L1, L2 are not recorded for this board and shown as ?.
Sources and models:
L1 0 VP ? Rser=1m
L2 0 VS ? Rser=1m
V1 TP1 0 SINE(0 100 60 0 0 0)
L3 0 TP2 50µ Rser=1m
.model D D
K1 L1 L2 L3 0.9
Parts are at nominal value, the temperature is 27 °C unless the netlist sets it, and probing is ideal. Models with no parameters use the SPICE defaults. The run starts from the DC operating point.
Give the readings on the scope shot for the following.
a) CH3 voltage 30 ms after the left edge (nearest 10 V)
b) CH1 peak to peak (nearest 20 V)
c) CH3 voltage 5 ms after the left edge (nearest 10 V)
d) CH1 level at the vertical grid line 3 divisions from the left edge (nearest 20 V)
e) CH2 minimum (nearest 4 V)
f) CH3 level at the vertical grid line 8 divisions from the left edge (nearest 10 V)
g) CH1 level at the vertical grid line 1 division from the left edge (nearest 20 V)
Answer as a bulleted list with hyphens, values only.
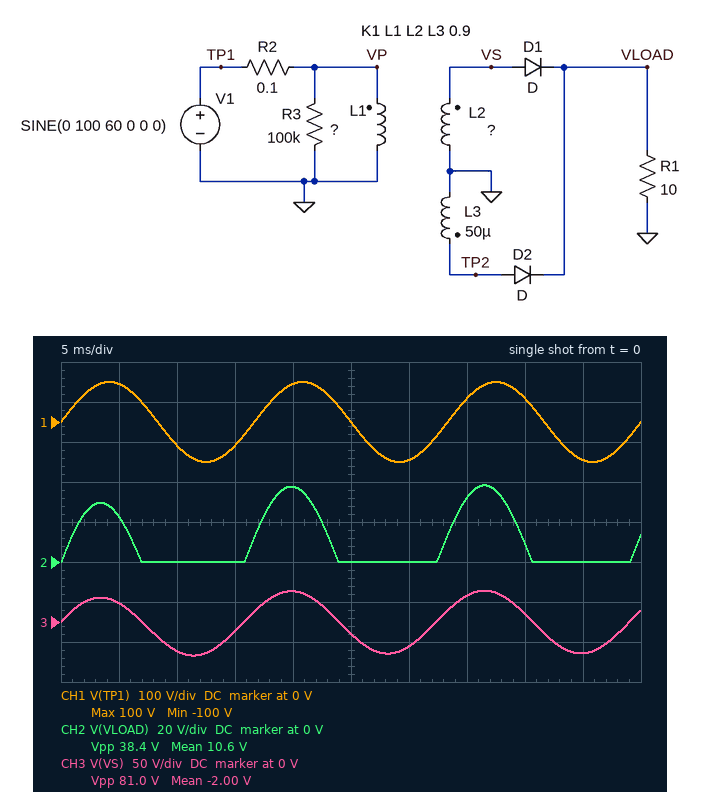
- -30 V
- 200 V
- 20 V
- -60 V
- 0 V
- 10 V
- 100 V
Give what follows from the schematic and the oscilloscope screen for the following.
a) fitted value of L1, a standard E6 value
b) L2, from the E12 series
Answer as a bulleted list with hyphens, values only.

- 680 µH
- 150 µH
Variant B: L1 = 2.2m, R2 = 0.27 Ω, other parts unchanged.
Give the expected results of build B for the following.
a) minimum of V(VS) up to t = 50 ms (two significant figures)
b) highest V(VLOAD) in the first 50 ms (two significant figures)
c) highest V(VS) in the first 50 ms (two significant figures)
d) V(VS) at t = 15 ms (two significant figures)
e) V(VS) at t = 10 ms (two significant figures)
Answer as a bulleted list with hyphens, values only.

- -24 V
- 21 V
- 22 V
- -8.0 V
- -20 V
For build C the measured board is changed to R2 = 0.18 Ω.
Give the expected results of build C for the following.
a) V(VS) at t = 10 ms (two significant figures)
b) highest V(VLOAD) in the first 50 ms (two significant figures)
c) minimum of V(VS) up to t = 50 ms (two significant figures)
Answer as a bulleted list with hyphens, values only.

- -34 V
- 34 V
- -36 V
